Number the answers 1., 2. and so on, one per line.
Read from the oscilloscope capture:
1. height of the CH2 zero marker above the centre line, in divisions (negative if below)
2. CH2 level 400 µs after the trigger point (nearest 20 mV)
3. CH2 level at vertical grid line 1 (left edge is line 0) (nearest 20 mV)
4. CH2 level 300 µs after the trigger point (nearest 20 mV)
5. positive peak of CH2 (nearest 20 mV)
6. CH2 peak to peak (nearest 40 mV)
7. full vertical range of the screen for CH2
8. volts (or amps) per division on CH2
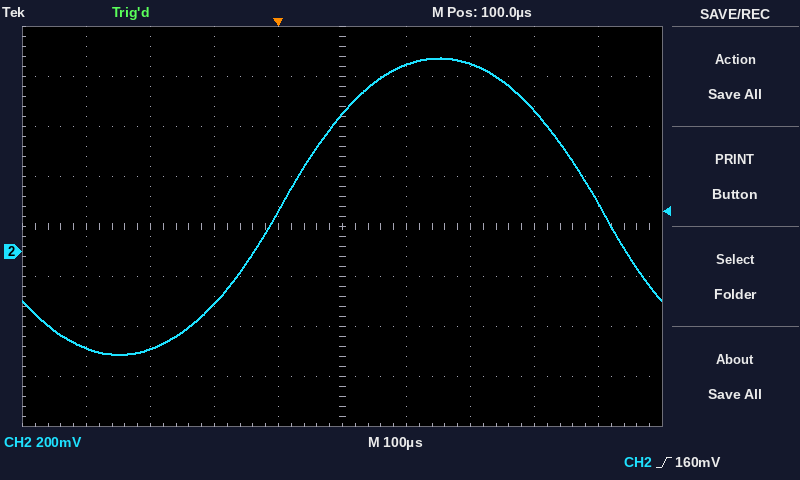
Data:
1. -0.5 div
2. 560 mV
3. -380 mV
4. 760 mV
5. 780 mV
6. 1.20 V
7. 1.6 V
8. 200 mV
